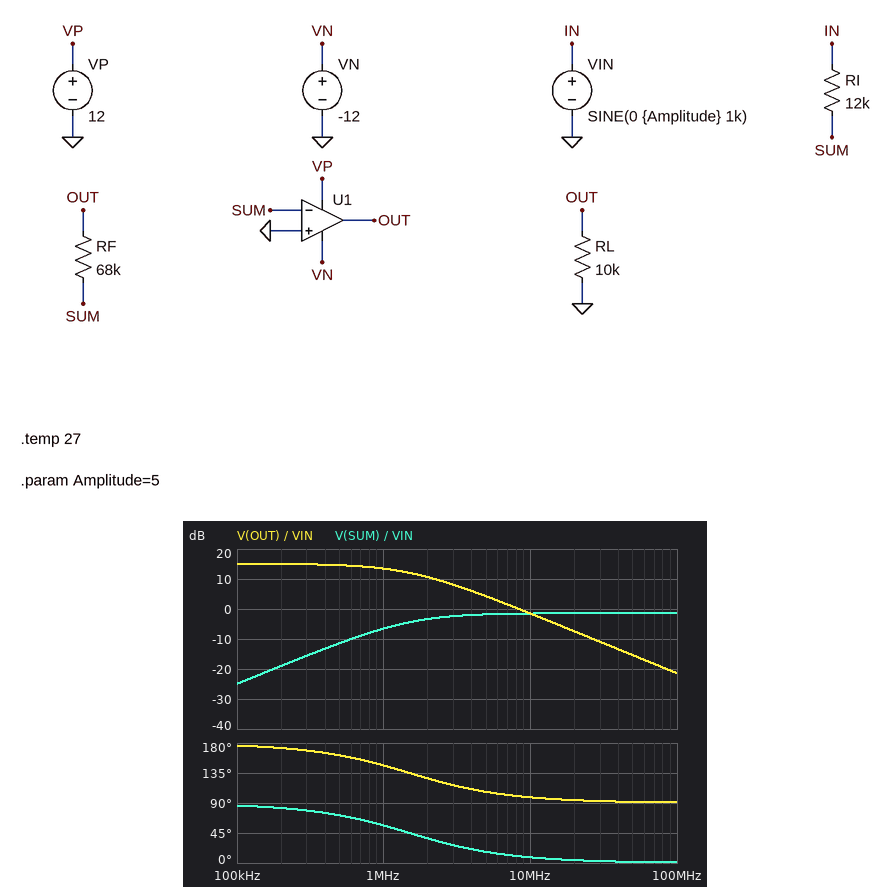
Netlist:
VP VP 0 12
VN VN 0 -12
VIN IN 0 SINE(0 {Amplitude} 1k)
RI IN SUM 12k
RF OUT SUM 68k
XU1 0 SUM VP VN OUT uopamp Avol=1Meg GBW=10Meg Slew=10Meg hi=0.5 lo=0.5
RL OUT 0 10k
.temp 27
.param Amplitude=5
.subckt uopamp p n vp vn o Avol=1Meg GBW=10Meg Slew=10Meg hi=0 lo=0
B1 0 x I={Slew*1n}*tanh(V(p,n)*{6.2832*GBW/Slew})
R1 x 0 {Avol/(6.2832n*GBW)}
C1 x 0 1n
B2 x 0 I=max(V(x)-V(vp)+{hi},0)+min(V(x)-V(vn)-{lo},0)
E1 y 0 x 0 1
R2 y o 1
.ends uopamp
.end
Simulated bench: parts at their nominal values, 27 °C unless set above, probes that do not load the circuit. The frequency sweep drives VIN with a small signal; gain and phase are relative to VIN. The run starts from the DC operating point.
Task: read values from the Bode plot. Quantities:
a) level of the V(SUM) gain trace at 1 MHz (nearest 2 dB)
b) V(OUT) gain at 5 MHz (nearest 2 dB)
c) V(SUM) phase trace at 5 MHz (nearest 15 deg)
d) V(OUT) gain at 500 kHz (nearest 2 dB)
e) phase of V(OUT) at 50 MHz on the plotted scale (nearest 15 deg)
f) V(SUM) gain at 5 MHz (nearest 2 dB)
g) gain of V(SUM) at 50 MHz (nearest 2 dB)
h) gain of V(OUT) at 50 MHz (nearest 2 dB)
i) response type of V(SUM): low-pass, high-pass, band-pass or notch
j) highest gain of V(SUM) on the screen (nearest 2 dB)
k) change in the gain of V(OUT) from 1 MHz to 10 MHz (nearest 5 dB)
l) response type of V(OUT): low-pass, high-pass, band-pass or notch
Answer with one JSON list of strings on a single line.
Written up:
["-6 dB", "4 dB", "15 deg", "14 dB", "90 deg", "-2 dB", "-2 dB", "-16 dB", "high-pass", "-2 dB", "-15 dB", "low-pass"]
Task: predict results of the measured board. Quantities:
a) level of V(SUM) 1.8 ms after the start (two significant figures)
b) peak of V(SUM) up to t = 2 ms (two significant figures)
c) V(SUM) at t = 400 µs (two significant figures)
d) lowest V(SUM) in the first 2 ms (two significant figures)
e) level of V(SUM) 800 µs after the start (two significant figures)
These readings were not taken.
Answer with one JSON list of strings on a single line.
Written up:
["-2.3 V", "2.5 V", "770 mV", "-2.5 V", "-2.3 V"]
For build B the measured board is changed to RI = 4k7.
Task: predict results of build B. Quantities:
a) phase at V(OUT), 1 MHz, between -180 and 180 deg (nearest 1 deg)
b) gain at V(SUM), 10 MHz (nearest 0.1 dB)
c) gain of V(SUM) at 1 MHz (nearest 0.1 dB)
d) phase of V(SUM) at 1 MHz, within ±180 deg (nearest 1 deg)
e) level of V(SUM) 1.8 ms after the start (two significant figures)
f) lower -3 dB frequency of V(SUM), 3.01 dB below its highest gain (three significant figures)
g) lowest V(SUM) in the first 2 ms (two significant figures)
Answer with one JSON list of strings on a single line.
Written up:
["123 deg", "-0.6 dB", "-2.1 dB", "33 deg", "-3.7 V", "646 kHz", "-3.9 V"]
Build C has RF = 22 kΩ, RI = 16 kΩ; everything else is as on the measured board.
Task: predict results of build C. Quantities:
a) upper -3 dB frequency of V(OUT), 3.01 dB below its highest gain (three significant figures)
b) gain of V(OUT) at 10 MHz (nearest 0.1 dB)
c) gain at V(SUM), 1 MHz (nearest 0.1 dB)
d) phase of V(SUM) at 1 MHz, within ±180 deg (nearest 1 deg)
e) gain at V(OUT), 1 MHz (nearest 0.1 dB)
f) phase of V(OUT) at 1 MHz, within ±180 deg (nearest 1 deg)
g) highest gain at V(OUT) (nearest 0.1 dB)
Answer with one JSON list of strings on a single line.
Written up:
["4.21 MHz", "-5.5 dB", "-17.5 dB", "77 deg", "2.5 dB", "167 deg", "2.8 dB"]
